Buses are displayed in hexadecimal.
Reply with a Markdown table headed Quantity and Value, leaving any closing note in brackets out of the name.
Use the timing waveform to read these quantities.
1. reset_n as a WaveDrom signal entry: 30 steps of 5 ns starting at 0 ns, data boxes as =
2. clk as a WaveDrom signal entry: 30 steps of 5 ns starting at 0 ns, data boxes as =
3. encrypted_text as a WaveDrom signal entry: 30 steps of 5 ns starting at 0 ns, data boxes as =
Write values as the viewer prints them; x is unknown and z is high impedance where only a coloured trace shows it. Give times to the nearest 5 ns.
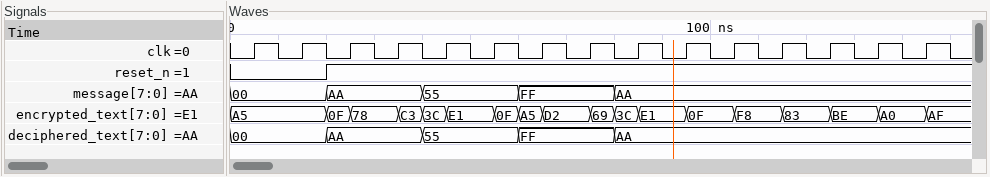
| Quantity | Value |
|---|---|
| reset_n as a WaveDrom signal entry: 30 steps of 5 ns starting at 0 ns, data boxes as = | {name: 'reset_n', wave: '0...1.........................'} |
| clk as a WaveDrom signal entry: 30 steps of 5 ns starting at 0 ns, data boxes as = | {name: 'clk', wave: '010101010101010101010101010101'} |
| encrypted_text as a WaveDrom signal entry: 30 steps of 5 ns starting at 0 ns, data boxes as = | {name: 'encrypted_text', wave: '=...==.===.===.===.=.=.=.=.=.=', data: 'A5 0F 78 C3 3C E1 0F A5 D2 69 3C E1 0F F8 83 BE A0 AF'} |
